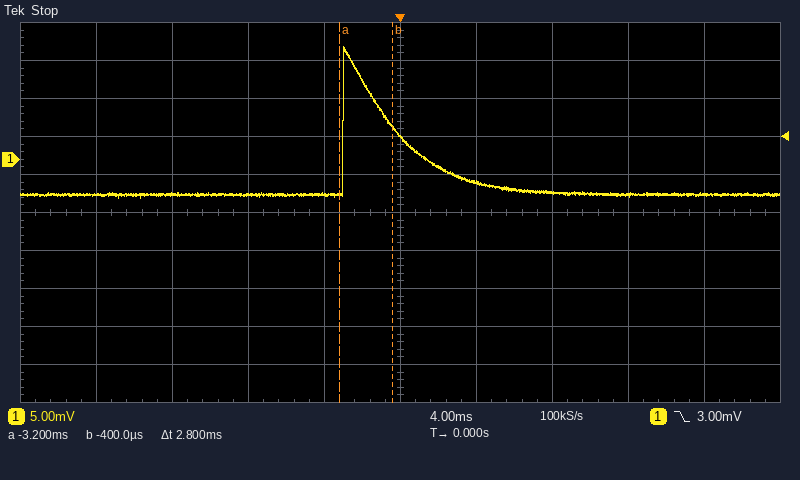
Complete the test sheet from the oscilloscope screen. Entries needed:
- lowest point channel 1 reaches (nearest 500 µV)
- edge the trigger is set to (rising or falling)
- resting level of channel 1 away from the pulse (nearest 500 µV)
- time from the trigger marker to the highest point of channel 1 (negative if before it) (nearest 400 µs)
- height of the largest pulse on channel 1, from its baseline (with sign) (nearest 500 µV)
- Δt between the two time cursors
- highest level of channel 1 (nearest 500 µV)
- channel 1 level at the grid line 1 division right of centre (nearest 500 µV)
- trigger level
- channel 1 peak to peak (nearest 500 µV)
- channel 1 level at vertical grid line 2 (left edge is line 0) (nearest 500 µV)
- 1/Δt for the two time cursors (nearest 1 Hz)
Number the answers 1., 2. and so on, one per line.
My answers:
1. -5.0 mV
2. falling
3. -4.5 mV
4. -2.8 ms
5. +19.5 mV
6. 2.8 ms
7. 15.0 mV
8. -3.0 mV
9. 3.00 mV
10. 20.0 mV
11. -4.5 mV
12. 357 Hz
